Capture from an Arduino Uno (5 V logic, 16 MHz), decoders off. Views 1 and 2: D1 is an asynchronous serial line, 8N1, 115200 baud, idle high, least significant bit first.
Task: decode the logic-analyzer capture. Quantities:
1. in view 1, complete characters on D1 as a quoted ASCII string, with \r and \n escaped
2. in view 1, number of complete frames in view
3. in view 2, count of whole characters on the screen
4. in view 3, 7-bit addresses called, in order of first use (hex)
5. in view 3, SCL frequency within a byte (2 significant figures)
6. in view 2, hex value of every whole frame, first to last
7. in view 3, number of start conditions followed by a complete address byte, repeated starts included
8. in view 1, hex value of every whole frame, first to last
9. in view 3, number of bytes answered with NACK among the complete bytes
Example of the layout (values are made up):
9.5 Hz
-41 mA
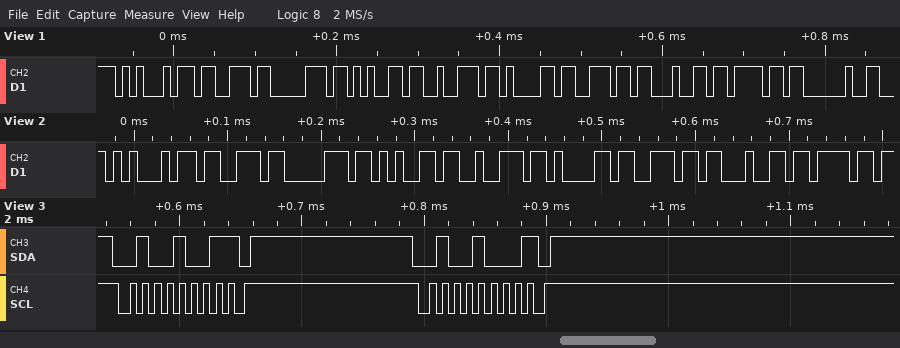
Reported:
"Esperando "
10
9
0x24
100 kHz
45 73 70 65 72 61 6E 64 6F
2
45 73 70 65 72 61 6E 64 6F 20
2
